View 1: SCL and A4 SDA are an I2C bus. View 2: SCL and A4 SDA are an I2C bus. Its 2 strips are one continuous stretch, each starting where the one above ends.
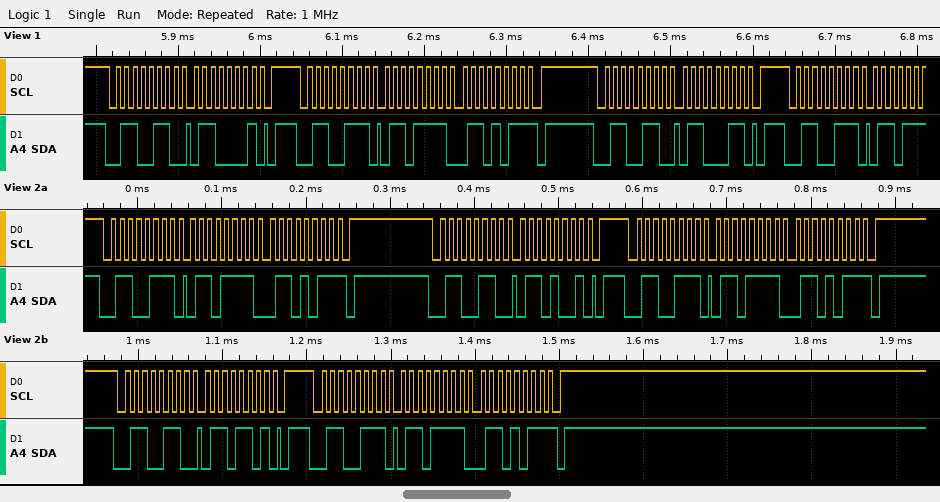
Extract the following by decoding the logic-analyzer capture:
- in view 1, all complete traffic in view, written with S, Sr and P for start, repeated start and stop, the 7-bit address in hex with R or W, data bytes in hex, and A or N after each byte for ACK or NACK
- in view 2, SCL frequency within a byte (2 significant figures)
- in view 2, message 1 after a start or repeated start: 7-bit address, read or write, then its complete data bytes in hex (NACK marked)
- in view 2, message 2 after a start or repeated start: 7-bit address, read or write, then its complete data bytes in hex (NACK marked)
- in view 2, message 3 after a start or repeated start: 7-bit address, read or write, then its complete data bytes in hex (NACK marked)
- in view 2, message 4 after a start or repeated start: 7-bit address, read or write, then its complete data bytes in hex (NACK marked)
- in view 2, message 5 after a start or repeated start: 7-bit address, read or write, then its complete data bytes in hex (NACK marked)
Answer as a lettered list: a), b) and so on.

a) S 33W A 61 A P S 33R A 6F A 6B N P S 33W A 63 A P S 33R A
b) 100 kHz
c) 0x33 read: 6F 6B NACK
d) 0x33 write: 69
e) 0x33 read: 6F 6B NACK
f) 0x33 write: 6D
g) 0x33 read: 6F 6B NACK
